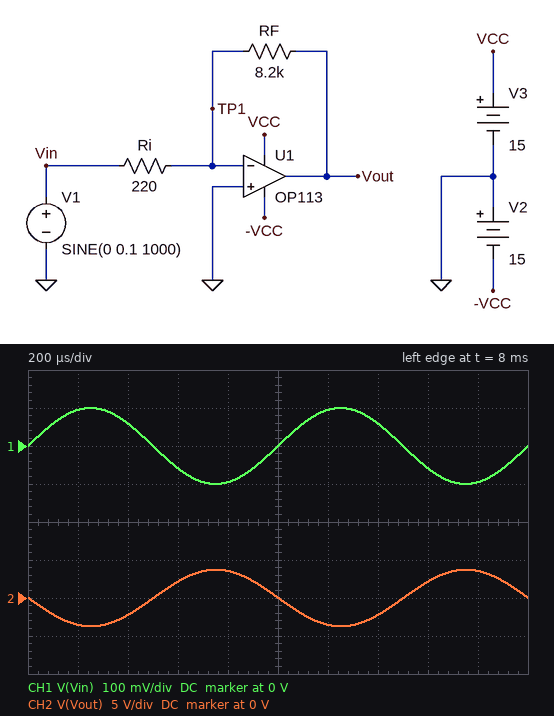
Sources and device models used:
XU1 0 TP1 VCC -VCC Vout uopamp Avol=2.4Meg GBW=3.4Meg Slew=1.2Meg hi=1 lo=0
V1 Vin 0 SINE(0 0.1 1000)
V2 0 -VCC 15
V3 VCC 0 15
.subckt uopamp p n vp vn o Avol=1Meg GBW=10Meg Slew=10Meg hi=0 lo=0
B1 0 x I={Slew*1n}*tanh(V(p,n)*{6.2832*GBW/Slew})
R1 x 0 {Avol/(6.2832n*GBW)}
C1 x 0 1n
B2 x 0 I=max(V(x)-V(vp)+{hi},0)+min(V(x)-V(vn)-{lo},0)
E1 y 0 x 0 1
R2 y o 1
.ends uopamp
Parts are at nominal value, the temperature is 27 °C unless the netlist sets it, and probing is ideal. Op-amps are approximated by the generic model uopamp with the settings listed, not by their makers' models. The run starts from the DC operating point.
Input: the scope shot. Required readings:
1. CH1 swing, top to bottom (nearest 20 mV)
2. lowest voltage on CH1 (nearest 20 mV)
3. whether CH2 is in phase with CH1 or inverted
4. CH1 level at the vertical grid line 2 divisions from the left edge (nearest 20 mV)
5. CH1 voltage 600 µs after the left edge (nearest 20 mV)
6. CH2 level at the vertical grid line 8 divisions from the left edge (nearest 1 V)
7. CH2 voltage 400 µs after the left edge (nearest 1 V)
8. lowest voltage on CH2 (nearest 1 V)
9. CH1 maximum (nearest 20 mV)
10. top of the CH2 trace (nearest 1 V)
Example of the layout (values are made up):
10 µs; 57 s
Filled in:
200 mV; -100 mV; inverted; 60 mV; -60 mV; 2 V; -2 V; -4 V; 100 mV; 4 V
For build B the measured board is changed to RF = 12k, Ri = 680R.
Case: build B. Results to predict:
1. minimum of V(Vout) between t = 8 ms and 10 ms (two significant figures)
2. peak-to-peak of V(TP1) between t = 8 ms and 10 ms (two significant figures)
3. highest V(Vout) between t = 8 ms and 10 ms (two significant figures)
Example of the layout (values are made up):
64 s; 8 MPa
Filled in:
-1.8 V; 1.0 mV; 1.8 V
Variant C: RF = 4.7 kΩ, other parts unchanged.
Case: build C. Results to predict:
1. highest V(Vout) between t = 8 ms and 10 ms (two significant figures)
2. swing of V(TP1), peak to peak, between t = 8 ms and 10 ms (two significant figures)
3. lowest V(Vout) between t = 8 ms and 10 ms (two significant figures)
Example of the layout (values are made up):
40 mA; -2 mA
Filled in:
2.1 V; 1.3 mV; -2.1 V
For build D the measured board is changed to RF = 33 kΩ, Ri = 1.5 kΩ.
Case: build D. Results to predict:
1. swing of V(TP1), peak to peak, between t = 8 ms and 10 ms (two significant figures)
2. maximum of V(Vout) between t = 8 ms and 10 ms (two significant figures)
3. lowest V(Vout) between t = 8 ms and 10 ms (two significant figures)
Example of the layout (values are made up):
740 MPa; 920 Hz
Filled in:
1.3 mV; 2.2 V; -2.2 V
